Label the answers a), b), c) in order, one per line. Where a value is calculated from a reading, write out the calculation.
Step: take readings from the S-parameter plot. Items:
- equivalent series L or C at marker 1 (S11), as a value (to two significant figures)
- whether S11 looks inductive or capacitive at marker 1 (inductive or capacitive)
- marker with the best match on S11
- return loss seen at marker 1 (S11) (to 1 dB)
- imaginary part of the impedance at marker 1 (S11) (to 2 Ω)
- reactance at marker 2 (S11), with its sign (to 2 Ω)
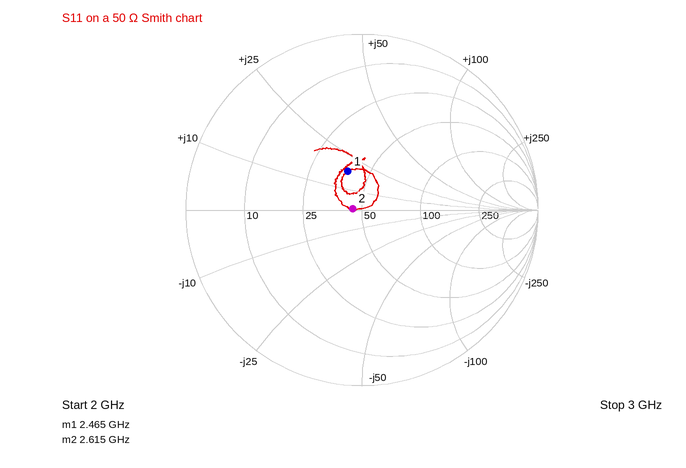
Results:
a) L = 18 Ω/(2π × 2.465 GHz) ≈ 1.2 nH
b) inductive
c) marker 2
d) 13 dB
e) +18 Ω
f) 0 Ω
